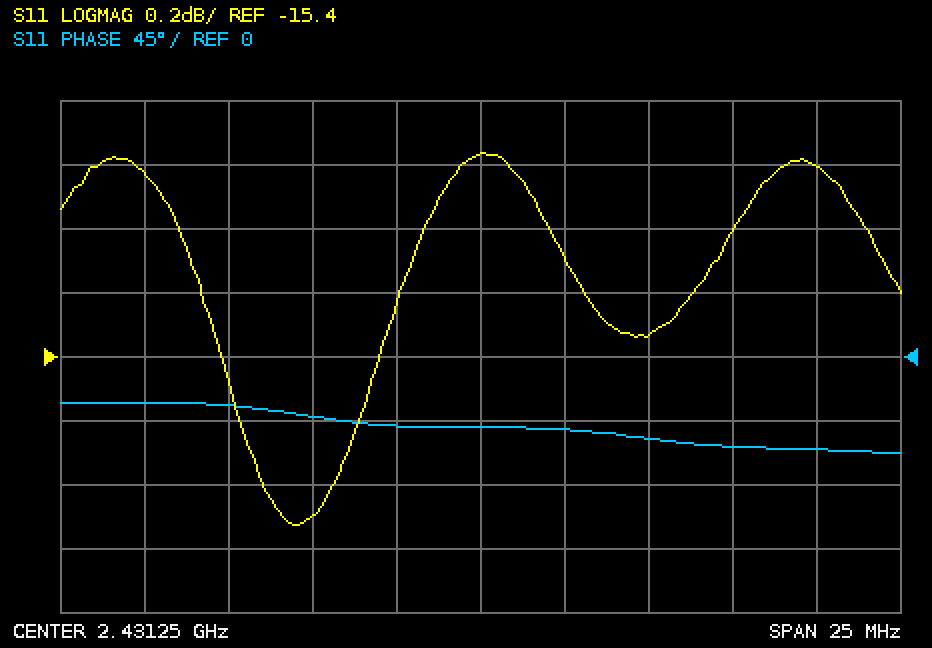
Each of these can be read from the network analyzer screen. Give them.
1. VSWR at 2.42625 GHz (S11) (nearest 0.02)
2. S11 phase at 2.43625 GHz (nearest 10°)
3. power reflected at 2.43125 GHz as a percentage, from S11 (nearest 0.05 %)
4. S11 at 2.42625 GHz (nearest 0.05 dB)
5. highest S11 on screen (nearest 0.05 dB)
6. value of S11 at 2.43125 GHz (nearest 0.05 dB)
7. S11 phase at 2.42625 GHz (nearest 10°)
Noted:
1.38
-60°
3.35 %
-15.90 dB
-14.75 dB
-14.75 dB
-40°
